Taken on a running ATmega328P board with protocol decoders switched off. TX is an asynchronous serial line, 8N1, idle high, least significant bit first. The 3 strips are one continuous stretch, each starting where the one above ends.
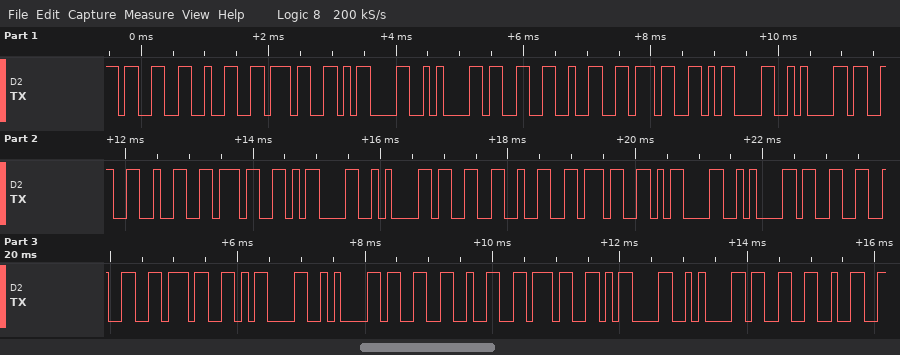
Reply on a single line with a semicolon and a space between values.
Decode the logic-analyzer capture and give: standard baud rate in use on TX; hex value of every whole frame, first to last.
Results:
9600 baud; 33 32 37 0D 0A 33 32 37 0D 0A 33 32 37 0D 0A 33 32 37 0D 0A 33 32 37 0D 0A 33 32 37 0D 0A 33 32
